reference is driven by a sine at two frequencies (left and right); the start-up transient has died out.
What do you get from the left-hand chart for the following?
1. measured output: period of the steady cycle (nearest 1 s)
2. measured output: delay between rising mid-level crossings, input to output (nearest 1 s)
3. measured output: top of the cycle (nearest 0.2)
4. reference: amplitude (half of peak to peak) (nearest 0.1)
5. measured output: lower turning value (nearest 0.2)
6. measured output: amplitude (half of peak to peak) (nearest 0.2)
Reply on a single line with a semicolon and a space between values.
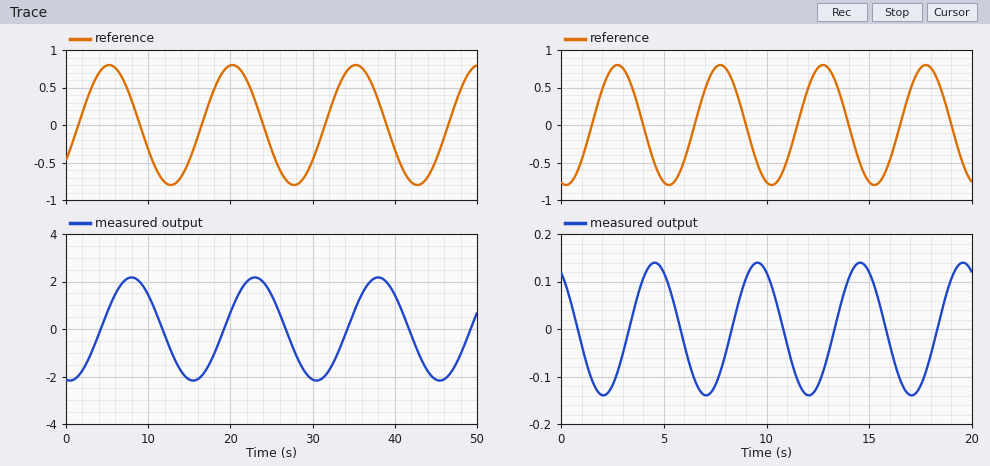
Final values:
15 s; 3 s; 2.2; 0.8; -2.2; 2.2
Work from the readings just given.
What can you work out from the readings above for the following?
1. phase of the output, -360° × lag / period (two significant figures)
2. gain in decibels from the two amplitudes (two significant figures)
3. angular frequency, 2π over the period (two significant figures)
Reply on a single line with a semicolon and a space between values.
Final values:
-72°; 8.8 dB; 0.42 rad/s
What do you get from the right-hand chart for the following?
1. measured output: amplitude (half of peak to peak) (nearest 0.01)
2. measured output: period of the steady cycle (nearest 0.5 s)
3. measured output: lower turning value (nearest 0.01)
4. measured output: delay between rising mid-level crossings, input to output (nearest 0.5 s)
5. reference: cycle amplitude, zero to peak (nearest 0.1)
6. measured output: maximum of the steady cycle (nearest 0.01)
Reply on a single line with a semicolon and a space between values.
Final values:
0.14; 5.0 s; -0.14; 2.0 s; 0.8; 0.14
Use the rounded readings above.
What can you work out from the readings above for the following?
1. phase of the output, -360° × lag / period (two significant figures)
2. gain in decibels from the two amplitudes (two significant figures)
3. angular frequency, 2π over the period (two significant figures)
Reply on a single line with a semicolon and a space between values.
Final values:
-140°; -15 dB; 1.3 rad/s
